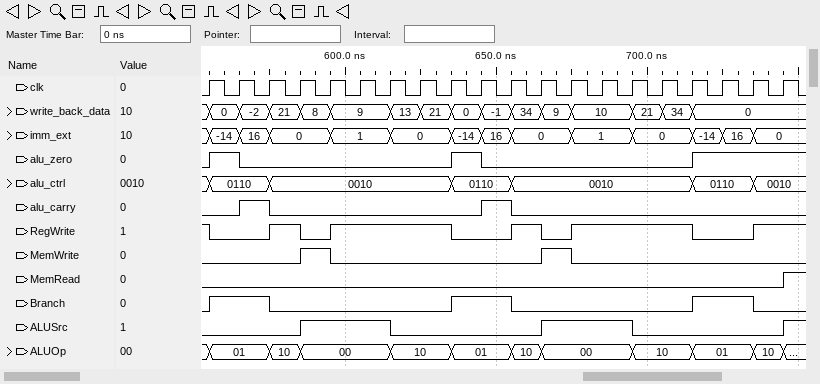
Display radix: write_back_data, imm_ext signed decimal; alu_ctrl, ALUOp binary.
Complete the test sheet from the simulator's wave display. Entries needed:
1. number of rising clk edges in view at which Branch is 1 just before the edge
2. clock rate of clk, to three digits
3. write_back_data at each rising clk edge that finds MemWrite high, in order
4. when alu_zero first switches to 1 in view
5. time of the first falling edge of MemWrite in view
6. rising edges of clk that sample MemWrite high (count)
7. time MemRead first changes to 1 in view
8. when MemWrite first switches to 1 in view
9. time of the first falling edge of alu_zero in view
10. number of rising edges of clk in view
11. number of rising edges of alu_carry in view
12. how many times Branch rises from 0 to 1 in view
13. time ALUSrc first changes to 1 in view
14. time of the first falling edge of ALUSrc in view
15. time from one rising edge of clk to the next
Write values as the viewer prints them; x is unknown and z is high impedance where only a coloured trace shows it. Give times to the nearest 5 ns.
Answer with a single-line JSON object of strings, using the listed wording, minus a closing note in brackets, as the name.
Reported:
{"number of rising clk edges in view at which Branch is 1 just before the edge": "6", "clock rate of clk, to three digits": "100 MHz", "write_back_data at each rising clk edge that finds MemWrite high, in order": "8, 9", "when alu_zero first switches to 1 in view": "555 ns", "time of the first falling edge of MemWrite in view": "595 ns", "rising edges of clk that sample MemWrite high": "2", "time MemRead first changes to 1 in view": "745 ns", "when MemWrite first switches to 1 in view": "585 ns", "time of the first falling edge of alu_zero in view": "565 ns", "number of rising edges of clk in view": "20", "number of rising edges of alu_carry in view": "2", "how many times Branch rises from 0 to 1 in view": "3", "time ALUSrc first changes to 1 in view": "585 ns", "time of the first falling edge of ALUSrc in view": "615 ns", "time from one rising edge of clk to the next": "10 ns"}
